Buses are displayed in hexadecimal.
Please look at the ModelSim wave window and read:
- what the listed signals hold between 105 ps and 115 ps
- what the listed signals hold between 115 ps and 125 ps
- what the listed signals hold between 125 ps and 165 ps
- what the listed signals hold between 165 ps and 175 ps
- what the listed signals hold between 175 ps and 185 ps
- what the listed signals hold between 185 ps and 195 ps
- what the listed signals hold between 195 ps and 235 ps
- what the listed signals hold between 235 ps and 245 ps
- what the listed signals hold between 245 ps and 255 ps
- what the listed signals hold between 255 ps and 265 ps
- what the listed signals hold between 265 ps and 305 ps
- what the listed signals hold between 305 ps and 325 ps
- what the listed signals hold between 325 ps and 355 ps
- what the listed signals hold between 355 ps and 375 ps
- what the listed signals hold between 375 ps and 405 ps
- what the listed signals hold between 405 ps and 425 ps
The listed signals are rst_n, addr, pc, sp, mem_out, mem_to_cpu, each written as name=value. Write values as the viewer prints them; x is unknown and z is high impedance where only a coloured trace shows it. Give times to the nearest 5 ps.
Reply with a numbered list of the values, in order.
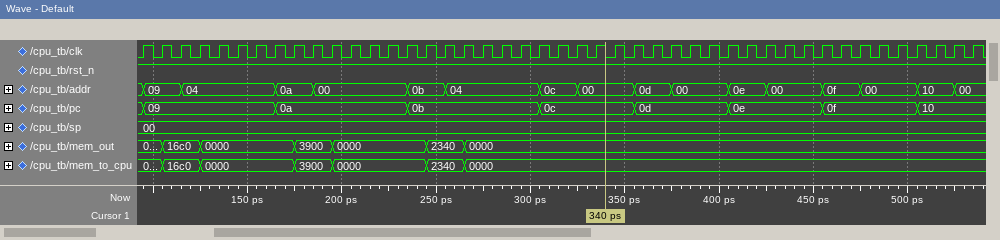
1. rst_n=1, addr=09, pc=09, sp=00, mem_out=16c0, mem_to_cpu=16c0
2. rst_n=1, addr=04, pc=09, sp=00, mem_out=16c0, mem_to_cpu=16c0
3. rst_n=1, addr=04, pc=09, sp=00, mem_out=0000, mem_to_cpu=0000
4. rst_n=1, addr=0a, pc=0a, sp=00, mem_out=0000, mem_to_cpu=0000
5. rst_n=1, addr=0a, pc=0a, sp=00, mem_out=3900, mem_to_cpu=3900
6. rst_n=1, addr=00, pc=0a, sp=00, mem_out=3900, mem_to_cpu=3900
7. rst_n=1, addr=00, pc=0a, sp=00, mem_out=0000, mem_to_cpu=0000
8. rst_n=1, addr=0b, pc=0b, sp=00, mem_out=0000, mem_to_cpu=0000
9. rst_n=1, addr=0b, pc=0b, sp=00, mem_out=2340, mem_to_cpu=2340
10. rst_n=1, addr=04, pc=0b, sp=00, mem_out=2340, mem_to_cpu=2340
11. rst_n=1, addr=04, pc=0b, sp=00, mem_out=0000, mem_to_cpu=0000
12. rst_n=1, addr=0c, pc=0c, sp=00, mem_out=0000, mem_to_cpu=0000
13. rst_n=1, addr=00, pc=0c, sp=00, mem_out=0000, mem_to_cpu=0000
14. rst_n=1, addr=0d, pc=0d, sp=00, mem_out=0000, mem_to_cpu=0000
15. rst_n=1, addr=00, pc=0d, sp=00, mem_out=0000, mem_to_cpu=0000
16. rst_n=1, addr=0e, pc=0e, sp=00, mem_out=0000, mem_to_cpu=0000
